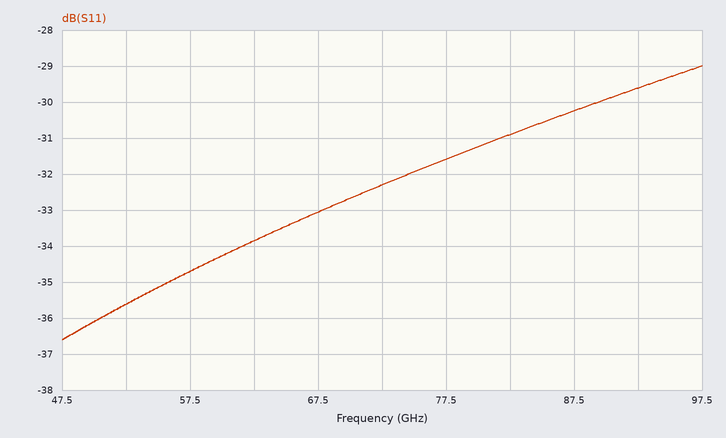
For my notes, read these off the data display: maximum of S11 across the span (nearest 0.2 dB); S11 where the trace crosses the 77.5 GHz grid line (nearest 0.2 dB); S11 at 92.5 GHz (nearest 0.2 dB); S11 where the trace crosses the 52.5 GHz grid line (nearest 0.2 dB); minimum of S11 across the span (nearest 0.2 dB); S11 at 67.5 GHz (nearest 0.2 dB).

-29.0 dB
-31.6 dB
-29.6 dB
-35.6 dB
-36.6 dB
-33.0 dB
